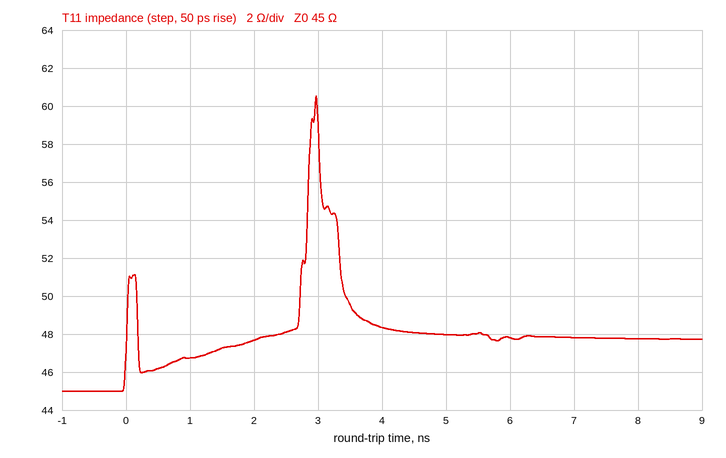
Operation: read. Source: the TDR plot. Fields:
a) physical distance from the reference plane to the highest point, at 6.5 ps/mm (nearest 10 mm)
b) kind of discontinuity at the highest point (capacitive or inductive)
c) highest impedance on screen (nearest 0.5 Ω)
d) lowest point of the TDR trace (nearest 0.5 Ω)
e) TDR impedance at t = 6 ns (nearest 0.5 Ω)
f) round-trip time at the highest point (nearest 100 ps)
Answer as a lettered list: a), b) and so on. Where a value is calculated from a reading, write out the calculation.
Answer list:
a) 3.0 ns / 2 / 6.5 ps/mm ≈ 231 mm, so 230 mm to the nearest 10 mm
b) inductive
c) 60.5 Ω
d) 45.0 Ω
e) 48.0 Ω
f) 3.0 ns
